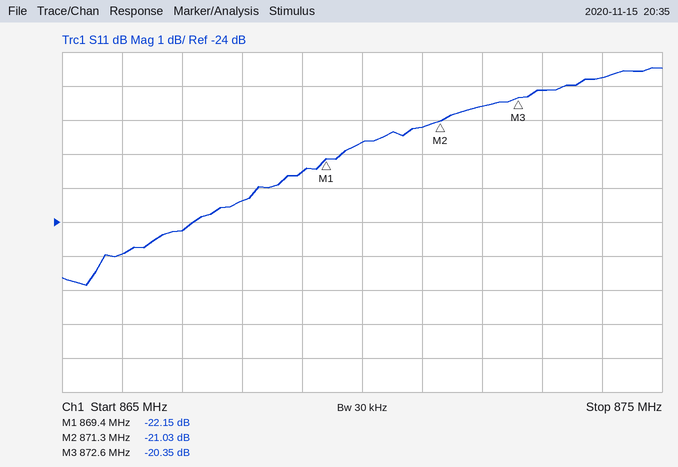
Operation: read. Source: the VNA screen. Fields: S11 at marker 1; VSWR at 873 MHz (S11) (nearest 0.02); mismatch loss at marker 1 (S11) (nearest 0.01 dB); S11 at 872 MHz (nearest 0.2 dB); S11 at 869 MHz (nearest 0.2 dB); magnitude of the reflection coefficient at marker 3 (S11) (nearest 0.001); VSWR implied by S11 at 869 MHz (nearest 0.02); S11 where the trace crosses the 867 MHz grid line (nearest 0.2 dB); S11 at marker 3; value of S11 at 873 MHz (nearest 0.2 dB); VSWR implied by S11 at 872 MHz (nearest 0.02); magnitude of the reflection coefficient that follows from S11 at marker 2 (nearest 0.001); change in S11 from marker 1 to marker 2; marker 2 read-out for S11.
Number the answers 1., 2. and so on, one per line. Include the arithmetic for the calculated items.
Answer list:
1. -22.15 dB
2. |Γ| = 10^(-20.2/20) = 0.0977; VSWR = (1 + 0.0977)/(1 − 0.0977) ≈ 1.22
3. −10 log10(1 − 10^(-22.15/10)) ≈ 0.03 dB
4. -20.6 dB
5. -22.6 dB
6. 10^(-20.35/20) ≈ 0.096
7. |Γ| = 10^(-22.6/20) = 0.0741; VSWR = (1 + 0.0741)/(1 − 0.0741) ≈ 1.16
8. -24.2 dB
9. -20.35 dB
10. -20.2 dB
11. |Γ| = 10^(-20.6/20) = 0.0933; VSWR = (1 + 0.0933)/(1 − 0.0933) ≈ 1.21, so 1.20 to the nearest 0.02
12. 10^(-21.03/20) ≈ 0.089
13. -21.03 − (-22.15) = 1.12 dB
14. -21.03 dB
